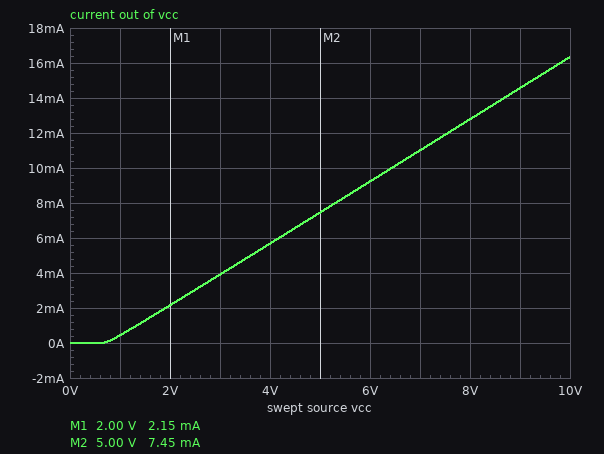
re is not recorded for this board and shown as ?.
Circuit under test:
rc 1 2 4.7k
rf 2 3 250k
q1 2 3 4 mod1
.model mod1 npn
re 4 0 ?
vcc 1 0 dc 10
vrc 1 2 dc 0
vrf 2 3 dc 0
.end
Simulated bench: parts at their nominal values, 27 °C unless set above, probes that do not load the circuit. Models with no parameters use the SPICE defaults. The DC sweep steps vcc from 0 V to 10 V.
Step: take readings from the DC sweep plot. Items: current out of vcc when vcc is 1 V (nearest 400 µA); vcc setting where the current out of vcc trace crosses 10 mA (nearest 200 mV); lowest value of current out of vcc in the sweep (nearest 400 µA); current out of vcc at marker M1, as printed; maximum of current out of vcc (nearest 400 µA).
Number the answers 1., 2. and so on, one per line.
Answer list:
1. 400 µA
2. 6.4 V
3. 0 A
4. 2.15 mA
5. 16.4 mA
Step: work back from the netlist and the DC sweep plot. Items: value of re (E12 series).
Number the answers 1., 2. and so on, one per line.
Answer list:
1. 560 Ω
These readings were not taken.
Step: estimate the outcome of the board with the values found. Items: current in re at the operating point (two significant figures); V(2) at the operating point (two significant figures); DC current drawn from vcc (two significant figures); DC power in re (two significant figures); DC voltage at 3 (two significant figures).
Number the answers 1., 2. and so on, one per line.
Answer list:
1. 16 mA
2. 10 V
3. 16 mA
4. 150 mW
5. 10 V
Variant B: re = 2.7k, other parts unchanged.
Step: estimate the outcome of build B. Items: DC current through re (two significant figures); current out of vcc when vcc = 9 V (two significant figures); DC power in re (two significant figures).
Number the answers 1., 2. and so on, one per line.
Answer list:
1. 3.4 mA
2. 3.0 mA
3. 31 mW
